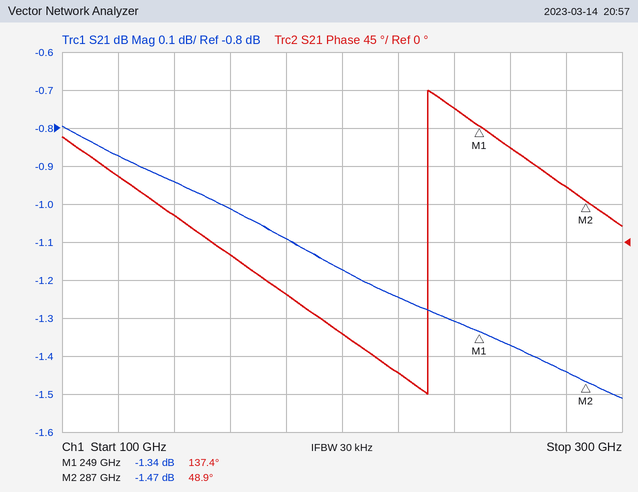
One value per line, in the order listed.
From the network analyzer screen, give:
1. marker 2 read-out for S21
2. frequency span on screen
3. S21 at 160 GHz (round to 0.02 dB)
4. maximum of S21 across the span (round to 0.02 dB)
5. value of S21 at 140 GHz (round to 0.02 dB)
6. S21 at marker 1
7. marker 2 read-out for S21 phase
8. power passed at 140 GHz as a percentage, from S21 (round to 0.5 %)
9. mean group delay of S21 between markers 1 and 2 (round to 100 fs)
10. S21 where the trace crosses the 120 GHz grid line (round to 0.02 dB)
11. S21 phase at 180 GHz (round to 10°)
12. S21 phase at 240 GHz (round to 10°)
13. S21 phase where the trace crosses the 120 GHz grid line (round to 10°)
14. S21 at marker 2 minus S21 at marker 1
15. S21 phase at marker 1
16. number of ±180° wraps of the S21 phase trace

-1.47 dB
200 GHz
-1.02 dB
-0.80 dB
-0.94 dB
-1.34 dB
48.9°
80.5 %
6.5 ps
-0.88 dB
-60°
160°
80°
-0.13 dB
137.4°
1
